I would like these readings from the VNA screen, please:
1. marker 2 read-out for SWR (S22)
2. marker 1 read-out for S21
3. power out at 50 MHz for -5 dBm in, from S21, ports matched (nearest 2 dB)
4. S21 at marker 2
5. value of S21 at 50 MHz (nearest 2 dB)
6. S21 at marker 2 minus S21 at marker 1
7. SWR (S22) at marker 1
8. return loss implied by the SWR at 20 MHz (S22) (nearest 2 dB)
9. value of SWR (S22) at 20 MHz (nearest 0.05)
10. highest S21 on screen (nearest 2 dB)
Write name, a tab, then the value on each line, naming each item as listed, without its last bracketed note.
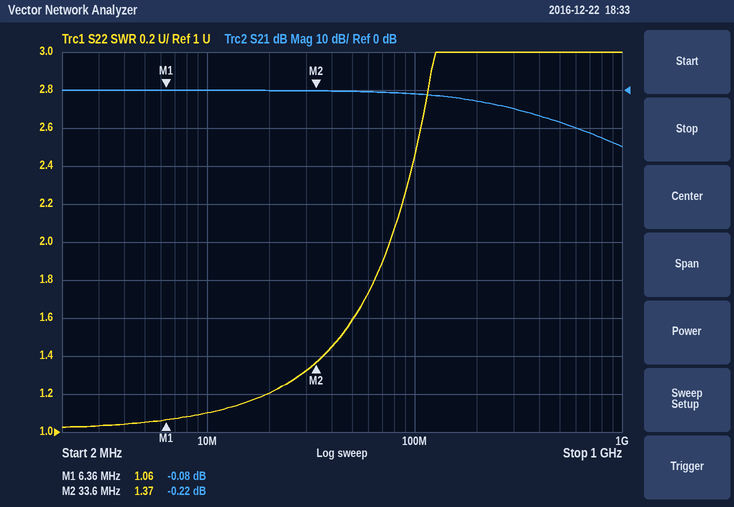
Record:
marker 2 read-out for SWR	1.37
marker 1 read-out for S21	-0.08 dB
power out at 50 MHz for -5 dBm in, from S21, ports matched	-6 dBm
S21 at marker 2	-0.22 dB
value of S21 at 50 MHz	0 dB
S21 at marker 2 minus S21 at marker 1	-0.14 dB
SWR (S22) at marker 1	1.06
return loss implied by the SWR at 20 MHz (S22)	20 dB
value of SWR (S22) at 20 MHz	1.20
highest S21 on screen	0 dB
